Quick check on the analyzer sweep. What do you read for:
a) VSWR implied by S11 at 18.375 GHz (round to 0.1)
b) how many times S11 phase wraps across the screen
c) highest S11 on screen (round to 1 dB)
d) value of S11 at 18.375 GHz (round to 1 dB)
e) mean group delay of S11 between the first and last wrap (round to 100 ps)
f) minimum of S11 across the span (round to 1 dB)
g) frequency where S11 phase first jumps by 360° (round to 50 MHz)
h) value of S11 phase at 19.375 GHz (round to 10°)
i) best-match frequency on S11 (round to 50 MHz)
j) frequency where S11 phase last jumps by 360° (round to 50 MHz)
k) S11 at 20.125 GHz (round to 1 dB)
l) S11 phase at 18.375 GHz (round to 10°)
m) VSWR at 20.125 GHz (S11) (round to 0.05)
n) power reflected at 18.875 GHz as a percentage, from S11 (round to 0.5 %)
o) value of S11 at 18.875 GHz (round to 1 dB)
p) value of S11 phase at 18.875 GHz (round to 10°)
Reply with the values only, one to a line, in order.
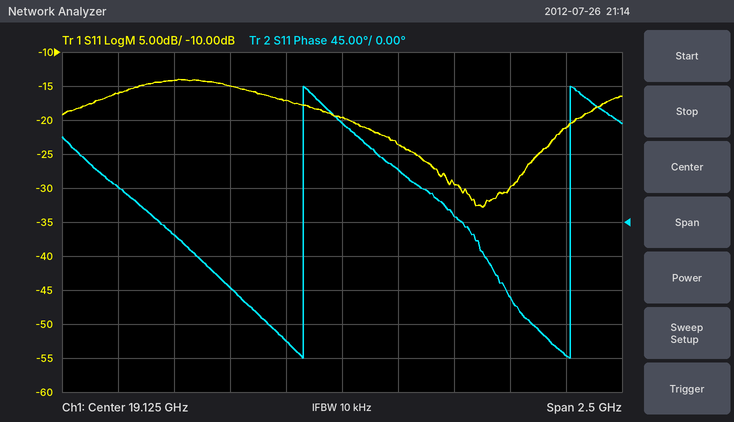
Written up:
1.5
2
-14 dB
-14 dB
800 ps
-33 dB
18.95 GHz
70°
19.75 GHz
20.15 GHz
-21 dB
-20°
1.20
2.0 %
-17 dB
-160°
